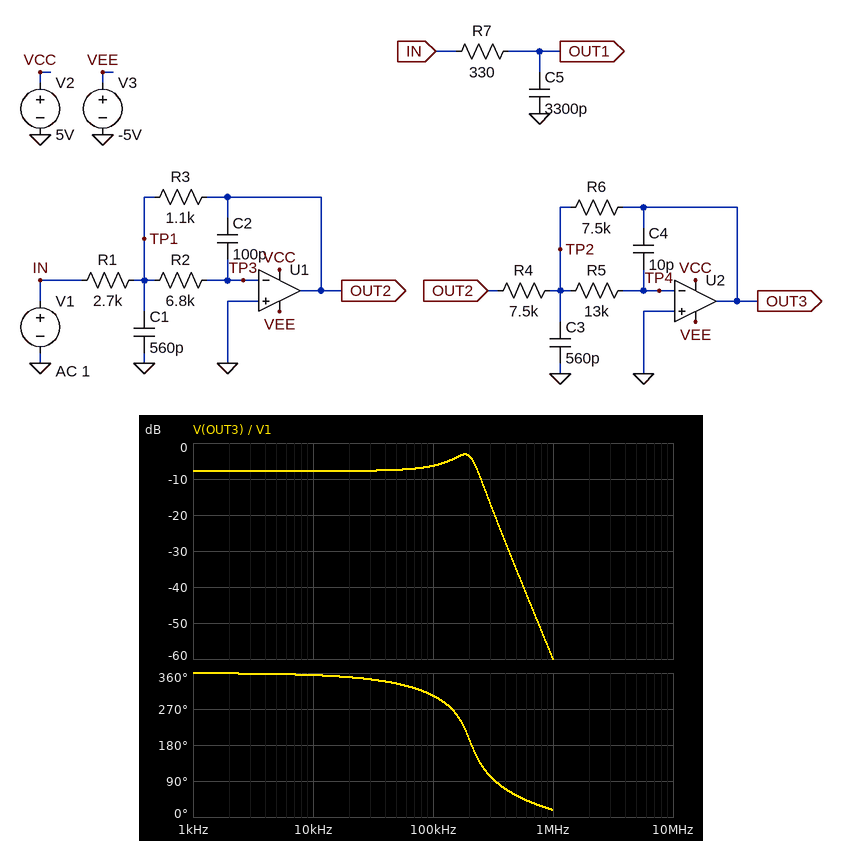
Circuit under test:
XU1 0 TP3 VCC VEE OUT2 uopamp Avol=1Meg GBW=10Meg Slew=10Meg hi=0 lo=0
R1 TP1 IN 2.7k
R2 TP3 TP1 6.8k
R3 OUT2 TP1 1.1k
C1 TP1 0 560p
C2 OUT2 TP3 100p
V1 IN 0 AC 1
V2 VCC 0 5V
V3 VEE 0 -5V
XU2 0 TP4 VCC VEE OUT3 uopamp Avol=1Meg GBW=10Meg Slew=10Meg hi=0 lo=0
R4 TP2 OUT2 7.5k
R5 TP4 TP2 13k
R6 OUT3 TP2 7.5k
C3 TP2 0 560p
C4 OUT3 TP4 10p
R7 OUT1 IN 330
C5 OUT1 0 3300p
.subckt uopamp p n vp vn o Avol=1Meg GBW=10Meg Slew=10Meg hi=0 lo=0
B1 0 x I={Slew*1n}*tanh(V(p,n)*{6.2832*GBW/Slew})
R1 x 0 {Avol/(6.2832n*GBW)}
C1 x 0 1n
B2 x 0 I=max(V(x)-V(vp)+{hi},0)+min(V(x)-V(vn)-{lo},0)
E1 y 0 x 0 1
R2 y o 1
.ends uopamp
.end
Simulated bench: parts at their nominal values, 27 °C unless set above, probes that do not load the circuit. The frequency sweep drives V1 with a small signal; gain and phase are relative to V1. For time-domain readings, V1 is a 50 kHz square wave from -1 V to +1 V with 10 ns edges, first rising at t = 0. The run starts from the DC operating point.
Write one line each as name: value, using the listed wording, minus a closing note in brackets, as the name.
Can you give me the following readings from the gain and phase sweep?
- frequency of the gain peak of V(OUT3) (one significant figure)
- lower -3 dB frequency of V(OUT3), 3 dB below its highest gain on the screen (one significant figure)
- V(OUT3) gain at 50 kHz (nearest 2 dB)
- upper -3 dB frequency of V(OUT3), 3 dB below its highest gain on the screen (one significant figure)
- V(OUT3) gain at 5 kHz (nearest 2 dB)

frequency of the gain peak of V(OUT3): 200 kHz
lower -3 dB frequency of V(OUT3), 3 dB below its highest gain on the screen: 100 kHz
V(OUT3) gain at 50 kHz: -8 dB
upper -3 dB frequency of V(OUT3), 3 dB below its highest gain on the screen: 200 kHz
V(OUT3) gain at 5 kHz: -8 dB
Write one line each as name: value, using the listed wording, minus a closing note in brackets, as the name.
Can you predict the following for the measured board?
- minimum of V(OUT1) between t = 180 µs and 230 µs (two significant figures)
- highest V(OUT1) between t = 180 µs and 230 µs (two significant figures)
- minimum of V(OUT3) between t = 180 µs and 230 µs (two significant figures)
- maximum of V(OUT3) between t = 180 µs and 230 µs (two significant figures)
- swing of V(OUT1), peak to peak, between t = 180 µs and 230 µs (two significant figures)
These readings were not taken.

minimum of V(OUT1) between t = 180 µs and 230 µs: -1.0 V
highest V(OUT1) between t = 180 µs and 230 µs: 1.0 V
minimum of V(OUT3) between t = 180 µs and 230 µs: -670 mV
maximum of V(OUT3) between t = 180 µs and 230 µs: 670 mV
swing of V(OUT1), peak to peak, between t = 180 µs and 230 µs: 2.0 V
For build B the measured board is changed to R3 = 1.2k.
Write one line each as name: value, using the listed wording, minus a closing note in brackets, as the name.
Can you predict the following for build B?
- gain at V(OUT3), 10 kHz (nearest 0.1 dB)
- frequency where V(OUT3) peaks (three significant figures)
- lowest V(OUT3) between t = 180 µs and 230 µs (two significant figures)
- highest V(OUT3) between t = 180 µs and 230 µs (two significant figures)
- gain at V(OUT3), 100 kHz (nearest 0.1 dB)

gain at V(OUT3), 10 kHz: -7.0 dB
frequency where V(OUT3) peaks: 184 kHz
lowest V(OUT3) between t = 180 µs and 230 µs: -730 mV
highest V(OUT3) between t = 180 µs and 230 µs: 730 mV
gain at V(OUT3), 100 kHz: -5.6 dB
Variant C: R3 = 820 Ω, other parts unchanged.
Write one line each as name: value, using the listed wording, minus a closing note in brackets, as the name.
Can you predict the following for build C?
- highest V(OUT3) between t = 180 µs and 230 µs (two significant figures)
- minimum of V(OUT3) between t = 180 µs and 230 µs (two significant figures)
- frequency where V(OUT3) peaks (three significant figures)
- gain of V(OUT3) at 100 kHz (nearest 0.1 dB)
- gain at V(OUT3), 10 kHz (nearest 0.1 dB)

highest V(OUT3) between t = 180 µs and 230 µs: 510 mV
minimum of V(OUT3) between t = 180 µs and 230 µs: -510 mV
frequency where V(OUT3) peaks: 186 kHz
gain of V(OUT3) at 100 kHz: -8.9 dB
gain at V(OUT3), 10 kHz: -10.3 dB
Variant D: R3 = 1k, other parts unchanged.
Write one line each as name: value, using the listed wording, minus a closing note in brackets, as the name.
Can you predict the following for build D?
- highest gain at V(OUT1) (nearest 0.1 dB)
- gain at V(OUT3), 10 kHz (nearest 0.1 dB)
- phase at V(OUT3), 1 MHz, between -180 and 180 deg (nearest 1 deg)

highest gain at V(OUT1): 0 dB
gain at V(OUT3), 10 kHz: -8.6 dB
phase at V(OUT3), 1 MHz, between -180 and 180 deg: 19 deg
